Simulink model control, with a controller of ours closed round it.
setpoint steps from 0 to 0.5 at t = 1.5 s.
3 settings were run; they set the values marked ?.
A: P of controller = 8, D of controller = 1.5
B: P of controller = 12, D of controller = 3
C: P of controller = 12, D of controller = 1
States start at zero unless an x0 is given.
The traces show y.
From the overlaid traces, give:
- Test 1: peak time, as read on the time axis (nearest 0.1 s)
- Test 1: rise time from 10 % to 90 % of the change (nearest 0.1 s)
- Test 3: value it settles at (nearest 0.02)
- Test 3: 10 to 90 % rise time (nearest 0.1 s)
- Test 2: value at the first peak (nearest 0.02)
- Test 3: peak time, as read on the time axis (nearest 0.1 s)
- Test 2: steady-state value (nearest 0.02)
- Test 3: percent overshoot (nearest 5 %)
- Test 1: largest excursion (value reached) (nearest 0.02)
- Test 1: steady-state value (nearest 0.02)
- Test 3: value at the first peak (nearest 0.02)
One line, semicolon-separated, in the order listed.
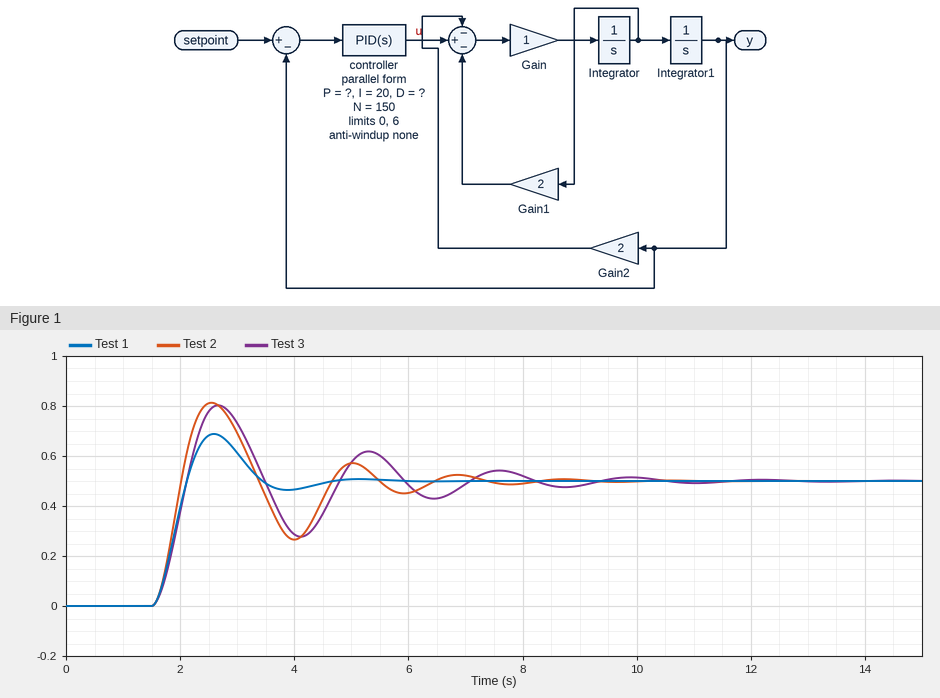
2.6 s; 0.4 s; 0.50; 0.4 s; 0.82; 2.7 s; 0.50; 60 %; 0.68; 0.50; 0.80
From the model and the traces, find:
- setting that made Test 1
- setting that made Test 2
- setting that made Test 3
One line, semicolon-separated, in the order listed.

B; C; A
